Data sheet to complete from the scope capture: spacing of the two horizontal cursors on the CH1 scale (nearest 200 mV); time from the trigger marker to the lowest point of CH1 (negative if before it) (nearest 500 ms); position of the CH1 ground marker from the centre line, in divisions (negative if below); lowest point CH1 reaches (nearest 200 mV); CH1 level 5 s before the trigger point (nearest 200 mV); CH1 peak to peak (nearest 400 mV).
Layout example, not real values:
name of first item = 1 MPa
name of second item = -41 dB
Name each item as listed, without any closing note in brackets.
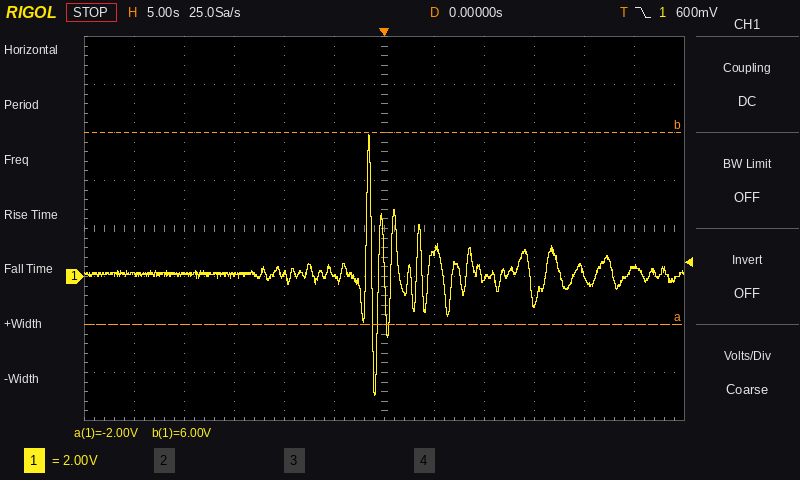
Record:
spacing of the two horizontal cursors on the CH1 scale = 8.0 V
time from the trigger marker to the lowest point of CH1 (negative if before it) = -1.0 s
position of the CH1 ground marker from the centre line, in divisions = -1.0 div
lowest point CH1 reaches = -5.0 V
CH1 level 5 s before the trigger point = 0.0 V
CH1 peak to peak = 10.8 V
